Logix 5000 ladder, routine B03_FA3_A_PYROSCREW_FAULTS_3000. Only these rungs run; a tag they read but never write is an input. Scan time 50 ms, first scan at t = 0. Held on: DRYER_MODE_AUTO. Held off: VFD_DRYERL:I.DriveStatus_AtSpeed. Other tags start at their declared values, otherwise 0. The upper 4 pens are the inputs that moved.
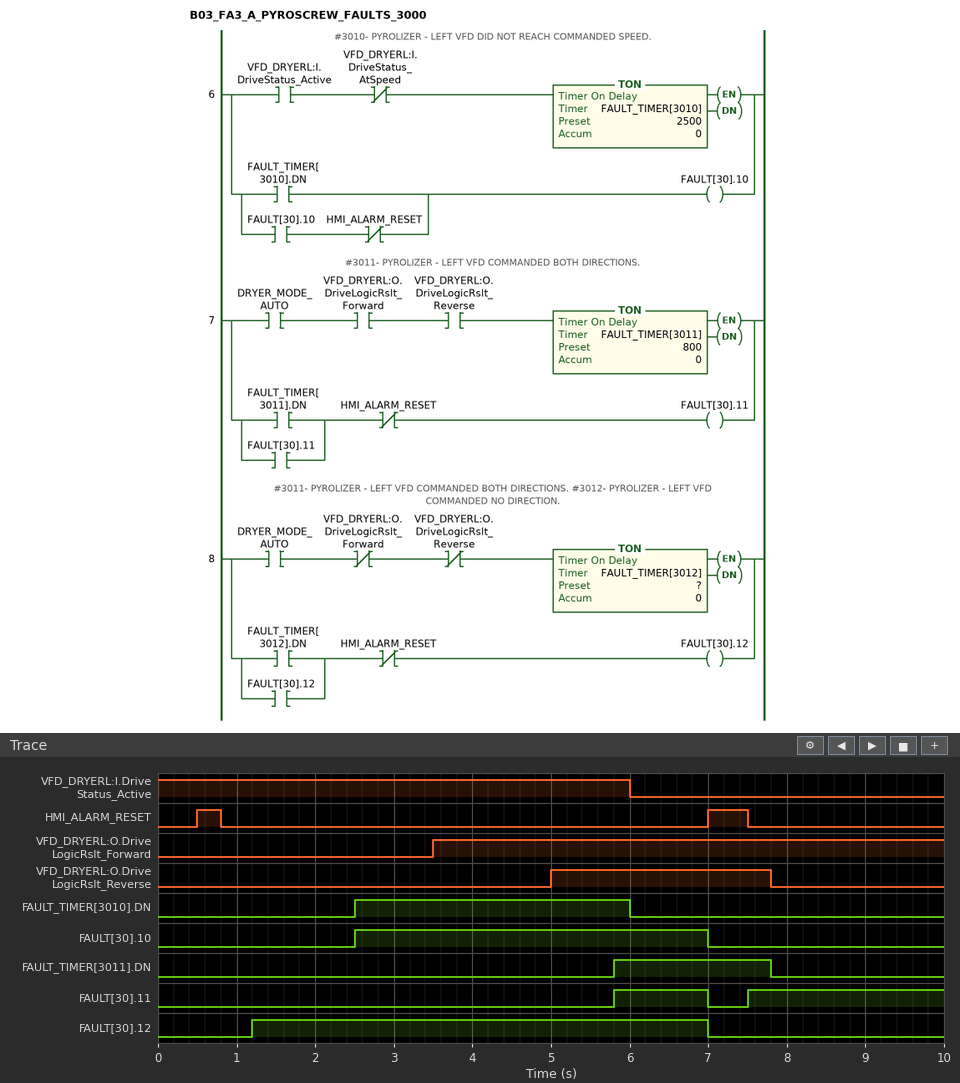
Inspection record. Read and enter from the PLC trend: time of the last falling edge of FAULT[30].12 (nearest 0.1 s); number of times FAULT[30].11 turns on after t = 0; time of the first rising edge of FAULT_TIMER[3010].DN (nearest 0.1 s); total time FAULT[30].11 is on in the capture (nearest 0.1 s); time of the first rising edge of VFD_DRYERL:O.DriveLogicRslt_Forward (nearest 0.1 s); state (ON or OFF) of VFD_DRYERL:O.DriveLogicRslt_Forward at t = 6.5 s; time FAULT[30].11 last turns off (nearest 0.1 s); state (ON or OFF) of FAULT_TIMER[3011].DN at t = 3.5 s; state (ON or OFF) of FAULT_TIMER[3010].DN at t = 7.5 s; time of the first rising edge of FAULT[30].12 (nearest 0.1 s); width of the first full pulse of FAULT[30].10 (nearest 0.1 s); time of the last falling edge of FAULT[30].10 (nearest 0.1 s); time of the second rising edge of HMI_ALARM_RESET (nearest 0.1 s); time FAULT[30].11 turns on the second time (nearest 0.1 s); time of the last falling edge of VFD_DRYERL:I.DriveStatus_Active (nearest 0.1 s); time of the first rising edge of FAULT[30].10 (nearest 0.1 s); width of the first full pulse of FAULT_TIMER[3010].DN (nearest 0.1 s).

7.0 s
2
2.5 s
3.7 s
3.5 s
ON
7.0 s
OFF
OFF
1.2 s
4.5 s
7.0 s
7.0 s
7.5 s
6.0 s
2.5 s
3.5 s
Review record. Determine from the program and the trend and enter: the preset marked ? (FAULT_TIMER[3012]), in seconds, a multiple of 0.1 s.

1.2 s
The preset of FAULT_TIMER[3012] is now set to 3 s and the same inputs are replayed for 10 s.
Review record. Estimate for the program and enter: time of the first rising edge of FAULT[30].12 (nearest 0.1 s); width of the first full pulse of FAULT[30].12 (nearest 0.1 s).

3.0 s
4.0 s
